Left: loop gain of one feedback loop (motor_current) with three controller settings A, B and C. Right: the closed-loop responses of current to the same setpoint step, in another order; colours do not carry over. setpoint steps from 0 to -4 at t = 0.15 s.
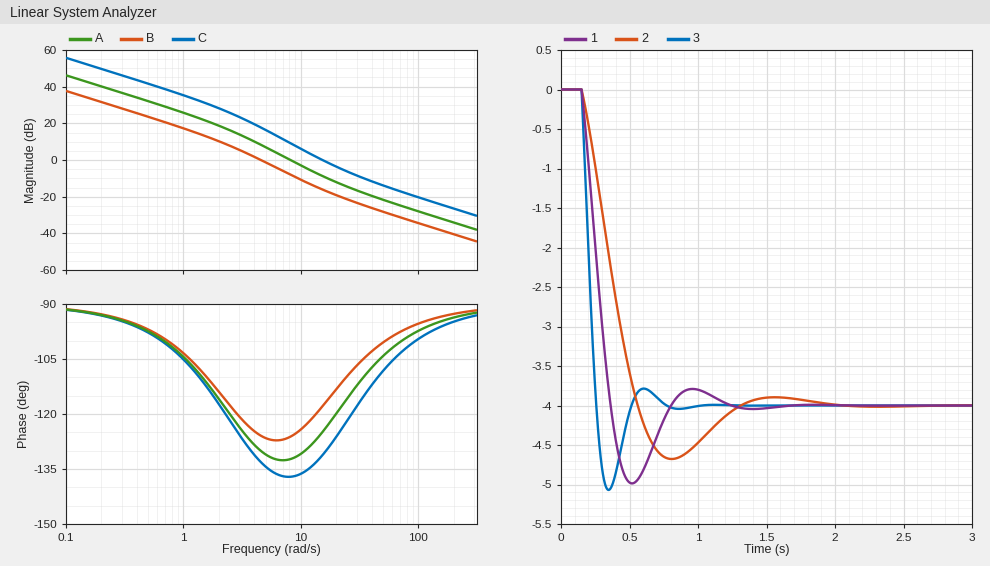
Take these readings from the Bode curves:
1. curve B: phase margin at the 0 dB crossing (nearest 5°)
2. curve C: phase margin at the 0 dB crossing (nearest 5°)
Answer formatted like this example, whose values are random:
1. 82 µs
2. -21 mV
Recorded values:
1. 55°
2. 50°
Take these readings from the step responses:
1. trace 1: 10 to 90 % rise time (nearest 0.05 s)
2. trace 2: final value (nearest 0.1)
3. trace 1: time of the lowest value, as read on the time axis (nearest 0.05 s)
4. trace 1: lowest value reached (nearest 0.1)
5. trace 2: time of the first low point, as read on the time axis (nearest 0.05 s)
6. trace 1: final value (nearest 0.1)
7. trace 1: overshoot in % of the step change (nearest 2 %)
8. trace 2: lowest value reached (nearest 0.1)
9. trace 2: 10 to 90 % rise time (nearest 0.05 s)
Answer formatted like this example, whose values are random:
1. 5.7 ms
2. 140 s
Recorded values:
1. 0.15 s
2. -4.0
3. 0.50 s
4. -5.0
5. 0.80 s
6. -4.0
7. 24 %
8. -4.7
9. 0.30 s
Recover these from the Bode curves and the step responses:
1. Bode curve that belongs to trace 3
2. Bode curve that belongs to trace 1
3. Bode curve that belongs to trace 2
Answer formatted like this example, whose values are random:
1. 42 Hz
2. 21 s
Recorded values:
1. C
2. A
3. B
